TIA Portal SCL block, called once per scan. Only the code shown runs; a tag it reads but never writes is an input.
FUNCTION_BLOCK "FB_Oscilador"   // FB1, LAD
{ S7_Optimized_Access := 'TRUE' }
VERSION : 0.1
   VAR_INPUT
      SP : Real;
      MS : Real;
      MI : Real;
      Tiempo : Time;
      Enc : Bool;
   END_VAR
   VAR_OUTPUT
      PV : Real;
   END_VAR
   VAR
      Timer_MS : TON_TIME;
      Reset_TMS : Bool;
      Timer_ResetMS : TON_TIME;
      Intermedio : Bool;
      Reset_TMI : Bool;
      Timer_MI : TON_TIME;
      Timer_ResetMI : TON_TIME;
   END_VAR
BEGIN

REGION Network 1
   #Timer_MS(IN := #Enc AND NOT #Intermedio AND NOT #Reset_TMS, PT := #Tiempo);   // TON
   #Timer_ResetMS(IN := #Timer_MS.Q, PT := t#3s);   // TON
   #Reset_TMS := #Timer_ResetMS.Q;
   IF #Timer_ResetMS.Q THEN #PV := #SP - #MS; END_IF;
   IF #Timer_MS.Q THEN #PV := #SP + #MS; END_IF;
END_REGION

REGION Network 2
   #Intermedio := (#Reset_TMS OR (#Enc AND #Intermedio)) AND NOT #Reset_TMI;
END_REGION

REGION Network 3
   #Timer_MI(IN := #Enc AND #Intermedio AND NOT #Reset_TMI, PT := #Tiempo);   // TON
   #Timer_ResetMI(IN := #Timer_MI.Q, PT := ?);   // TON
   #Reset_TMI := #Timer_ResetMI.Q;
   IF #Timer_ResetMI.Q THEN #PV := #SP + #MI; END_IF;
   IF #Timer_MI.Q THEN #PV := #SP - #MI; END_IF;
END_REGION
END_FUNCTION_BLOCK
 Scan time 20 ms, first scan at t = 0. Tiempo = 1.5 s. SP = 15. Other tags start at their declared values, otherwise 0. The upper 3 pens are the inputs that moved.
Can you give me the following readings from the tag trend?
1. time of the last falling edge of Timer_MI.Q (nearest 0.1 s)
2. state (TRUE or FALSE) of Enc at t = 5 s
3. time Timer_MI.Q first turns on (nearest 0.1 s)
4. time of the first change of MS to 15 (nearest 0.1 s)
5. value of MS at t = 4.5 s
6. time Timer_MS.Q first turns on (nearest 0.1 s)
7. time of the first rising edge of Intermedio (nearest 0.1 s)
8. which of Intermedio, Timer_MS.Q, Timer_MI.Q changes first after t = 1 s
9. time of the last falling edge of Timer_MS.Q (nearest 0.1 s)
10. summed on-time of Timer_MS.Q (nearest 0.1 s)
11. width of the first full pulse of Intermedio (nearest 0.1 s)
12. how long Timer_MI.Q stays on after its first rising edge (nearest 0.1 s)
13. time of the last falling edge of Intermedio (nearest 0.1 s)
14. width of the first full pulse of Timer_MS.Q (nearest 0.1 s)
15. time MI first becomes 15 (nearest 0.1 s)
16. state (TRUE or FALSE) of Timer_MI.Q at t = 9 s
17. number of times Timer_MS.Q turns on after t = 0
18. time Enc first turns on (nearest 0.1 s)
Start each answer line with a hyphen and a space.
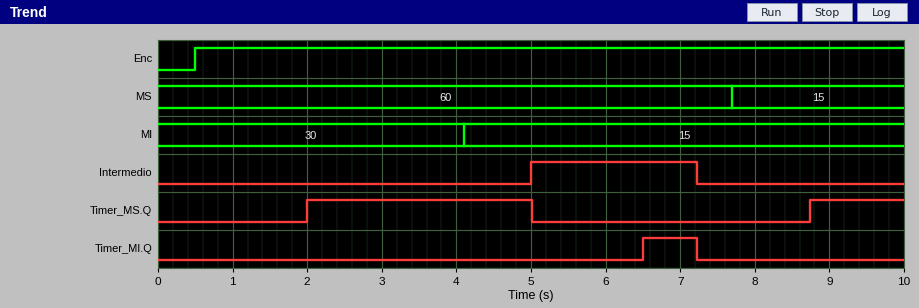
- 7.2 s
- TRUE
- 6.5 s
- 7.7 s
- 60
- 2.0 s
- 5.0 s
- Timer_MS.Q
- 5.0 s
- 4.3 s
- 2.2 s
- 0.7 s
- 7.2 s
- 3.0 s
- 4.1 s
- FALSE
- 2
- 0.5 s
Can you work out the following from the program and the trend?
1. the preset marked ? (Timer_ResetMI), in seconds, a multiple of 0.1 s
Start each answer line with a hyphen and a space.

- 0.7 s
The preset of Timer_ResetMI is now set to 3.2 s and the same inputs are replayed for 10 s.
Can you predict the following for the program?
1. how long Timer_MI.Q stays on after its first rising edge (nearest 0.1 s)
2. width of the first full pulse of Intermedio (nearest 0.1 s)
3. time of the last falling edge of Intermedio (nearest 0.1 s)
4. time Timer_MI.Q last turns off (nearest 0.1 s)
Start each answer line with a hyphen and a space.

- 3.2 s
- 4.7 s
- 9.7 s
- 9.7 s
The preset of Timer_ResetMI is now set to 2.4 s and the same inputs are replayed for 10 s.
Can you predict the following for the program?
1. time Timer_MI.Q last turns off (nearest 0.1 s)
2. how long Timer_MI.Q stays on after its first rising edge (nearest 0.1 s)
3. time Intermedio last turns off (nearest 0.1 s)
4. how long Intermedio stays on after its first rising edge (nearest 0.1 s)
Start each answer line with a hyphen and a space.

- 8.9 s
- 2.4 s
- 8.9 s
- 3.9 s
